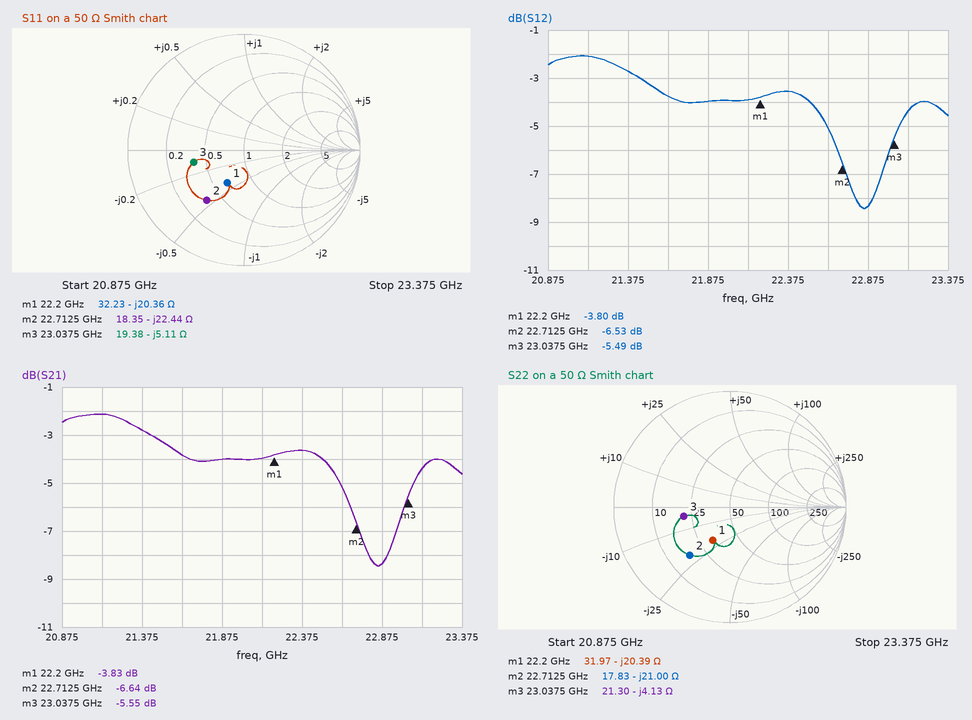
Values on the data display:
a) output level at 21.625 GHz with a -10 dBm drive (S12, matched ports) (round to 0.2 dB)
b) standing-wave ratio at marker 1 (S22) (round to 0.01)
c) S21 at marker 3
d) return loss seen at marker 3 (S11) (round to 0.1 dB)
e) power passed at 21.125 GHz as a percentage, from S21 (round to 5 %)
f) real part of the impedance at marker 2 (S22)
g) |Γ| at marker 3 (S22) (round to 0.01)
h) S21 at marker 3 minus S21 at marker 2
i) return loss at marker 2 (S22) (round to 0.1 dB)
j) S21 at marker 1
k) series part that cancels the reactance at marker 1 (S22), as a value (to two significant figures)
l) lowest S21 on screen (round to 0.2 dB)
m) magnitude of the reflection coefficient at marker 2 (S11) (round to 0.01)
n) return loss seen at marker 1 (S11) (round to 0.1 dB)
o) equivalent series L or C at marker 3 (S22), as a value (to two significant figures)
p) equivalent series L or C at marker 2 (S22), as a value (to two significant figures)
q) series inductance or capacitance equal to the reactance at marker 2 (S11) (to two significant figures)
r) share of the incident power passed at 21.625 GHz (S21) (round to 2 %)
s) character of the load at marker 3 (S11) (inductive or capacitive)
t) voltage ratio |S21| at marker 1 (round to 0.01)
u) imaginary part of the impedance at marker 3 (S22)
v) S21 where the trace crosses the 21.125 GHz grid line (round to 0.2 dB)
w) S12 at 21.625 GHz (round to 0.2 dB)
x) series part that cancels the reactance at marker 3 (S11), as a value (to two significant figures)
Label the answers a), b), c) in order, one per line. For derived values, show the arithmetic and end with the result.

a) -10 dBm + (-3.8 dB) = -13.8 dBm
b) 1.95
c) -5.55 dB
d) 7.0 dB
e) 10^(-2.2/10) ≈ 60 %
f) 17.83 Ω
g) 0.41
h) -5.55 − (-6.64) = 1.09 dB
i) 5.3 dB
j) -3.83 dB
k) L = 20.39 Ω/(2π × 22.2 GHz) ≈ 146 pH, so 150 pH to two significant figures
l) -8.4 dB
m) 0.54
n) 9.9 dB
o) C = 1/(2π × 23.0375 GHz × 4.13 Ω) ≈ 1.7 pF
p) C = 1/(2π × 22.7125 GHz × 21 Ω) ≈ 334 fF, so 330 fF to two significant figures
q) C = 1/(2π × 22.7125 GHz × 22.44 Ω) ≈ 312 fF, so 310 fF to two significant figures
r) 10^(-3.8/10) ≈ 42 %
s) capacitive
t) 10^(-3.83/20) ≈ 0.64
u) -4.13 Ω
v) -2.2 dB
w) -3.8 dB
x) L = 5.11 Ω/(2π × 23.0375 GHz) ≈ 35 pH
